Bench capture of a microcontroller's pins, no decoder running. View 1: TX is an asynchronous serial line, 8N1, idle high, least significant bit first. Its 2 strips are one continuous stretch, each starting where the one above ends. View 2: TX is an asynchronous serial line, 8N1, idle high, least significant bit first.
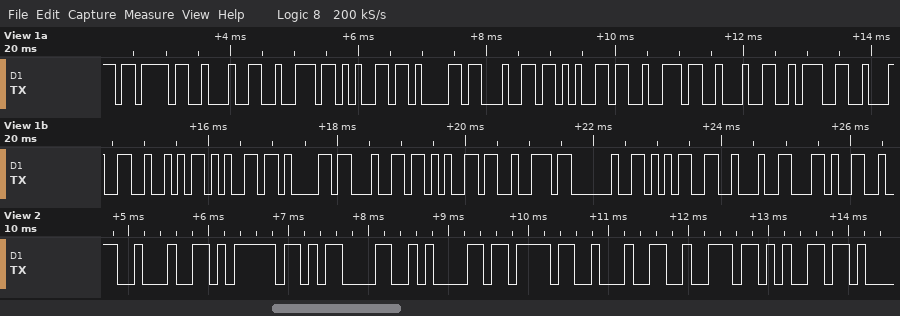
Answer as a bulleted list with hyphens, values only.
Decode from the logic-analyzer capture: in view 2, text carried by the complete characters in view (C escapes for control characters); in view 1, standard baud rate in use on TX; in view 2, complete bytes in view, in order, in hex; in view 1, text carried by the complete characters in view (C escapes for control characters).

- "\"}\r\n{\"re"
- 9600 baud
- 22 7D 0D 0A 7B 22 72 65
- "{\"reader\":\"Reader 5\","
